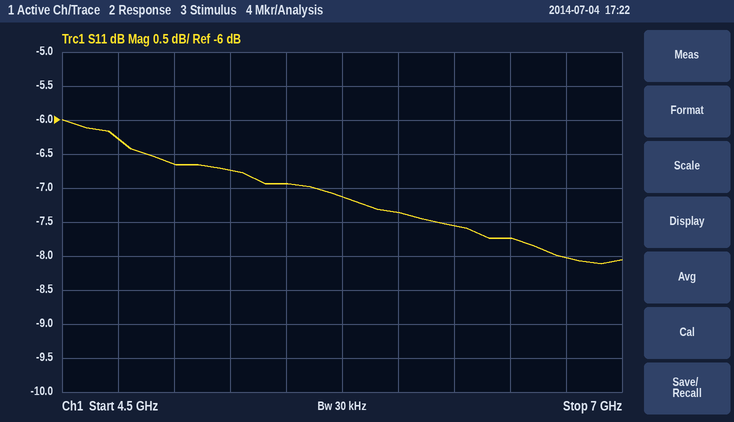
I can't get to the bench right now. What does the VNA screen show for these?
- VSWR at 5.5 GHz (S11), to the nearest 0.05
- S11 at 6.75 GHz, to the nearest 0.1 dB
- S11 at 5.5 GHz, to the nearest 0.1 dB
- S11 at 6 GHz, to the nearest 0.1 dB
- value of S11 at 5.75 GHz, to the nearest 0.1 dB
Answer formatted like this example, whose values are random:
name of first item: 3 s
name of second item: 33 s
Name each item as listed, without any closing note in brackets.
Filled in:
VSWR at 5.5 GHz (S11), to the nearest 0.05: 2.65
S11 at 6.75 GHz, to the nearest 0.1 dB: -8.0 dB
S11 at 5.5 GHz, to the nearest 0.1 dB: -6.9 dB
S11 at 6 GHz, to the nearest 0.1 dB: -7.4 dB
value of S11 at 5.75 GHz, to the nearest 0.1 dB: -7.1 dB
